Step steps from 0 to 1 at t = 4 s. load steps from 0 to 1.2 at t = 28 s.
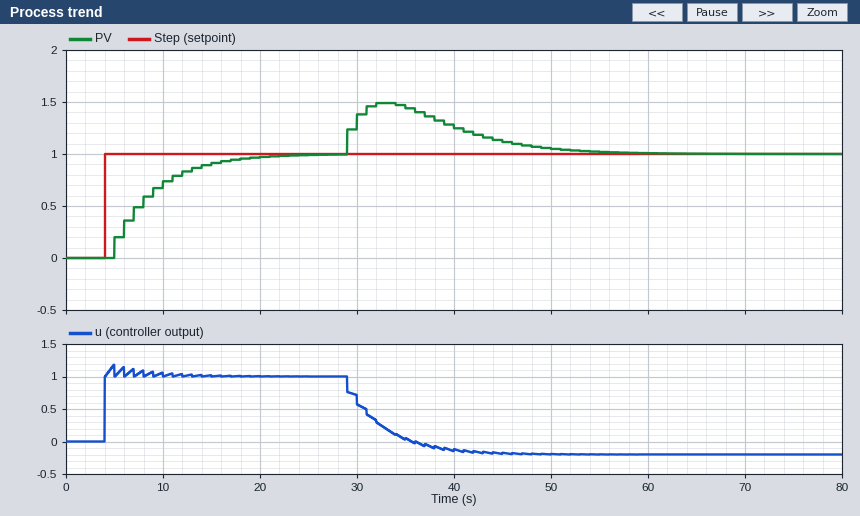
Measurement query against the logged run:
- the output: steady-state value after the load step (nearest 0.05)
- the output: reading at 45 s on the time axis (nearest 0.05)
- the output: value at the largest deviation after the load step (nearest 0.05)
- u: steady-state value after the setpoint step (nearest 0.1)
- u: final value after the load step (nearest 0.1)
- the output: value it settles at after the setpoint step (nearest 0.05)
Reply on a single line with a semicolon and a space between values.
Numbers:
1.00; 1.10; 1.50; 1.0; -0.2; 1.00
